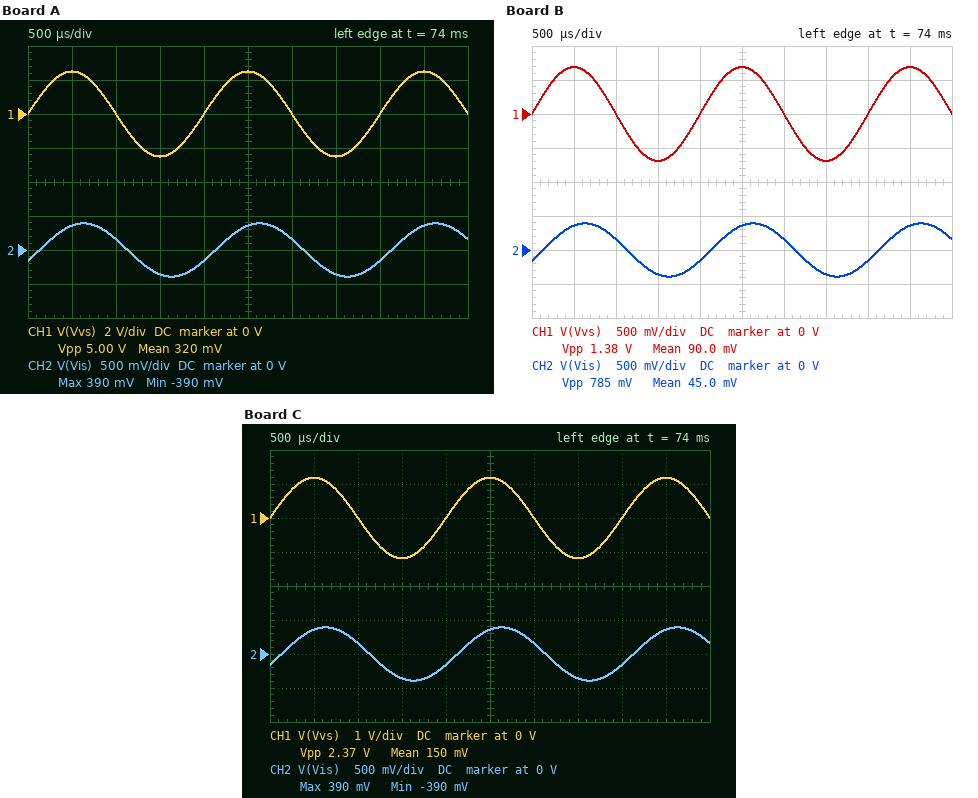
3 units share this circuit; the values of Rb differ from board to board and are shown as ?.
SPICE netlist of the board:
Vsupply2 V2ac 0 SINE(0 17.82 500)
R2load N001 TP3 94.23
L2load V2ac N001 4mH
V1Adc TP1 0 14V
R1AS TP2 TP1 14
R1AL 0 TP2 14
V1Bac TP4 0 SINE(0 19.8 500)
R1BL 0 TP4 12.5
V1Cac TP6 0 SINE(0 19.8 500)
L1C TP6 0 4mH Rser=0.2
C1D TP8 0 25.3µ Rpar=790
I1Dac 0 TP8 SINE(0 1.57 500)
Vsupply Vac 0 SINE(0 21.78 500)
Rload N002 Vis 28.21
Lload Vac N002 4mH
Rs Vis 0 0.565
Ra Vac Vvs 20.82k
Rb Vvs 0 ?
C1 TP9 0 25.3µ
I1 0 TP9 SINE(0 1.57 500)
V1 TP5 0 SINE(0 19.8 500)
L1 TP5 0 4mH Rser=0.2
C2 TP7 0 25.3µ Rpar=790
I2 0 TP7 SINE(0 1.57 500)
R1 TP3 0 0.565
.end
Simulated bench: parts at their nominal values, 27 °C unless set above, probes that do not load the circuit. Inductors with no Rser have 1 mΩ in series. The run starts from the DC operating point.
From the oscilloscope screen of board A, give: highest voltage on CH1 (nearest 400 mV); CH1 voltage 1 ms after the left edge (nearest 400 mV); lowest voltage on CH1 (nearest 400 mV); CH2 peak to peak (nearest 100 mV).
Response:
2.4 V
0 V
-2.4 V
800 mV
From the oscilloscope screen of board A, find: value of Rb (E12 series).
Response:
2.7 kΩ
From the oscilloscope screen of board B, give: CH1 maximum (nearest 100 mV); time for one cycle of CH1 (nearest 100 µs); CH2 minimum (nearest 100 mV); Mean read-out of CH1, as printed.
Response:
700 mV
2.0 ms
-400 mV
90.0 mV
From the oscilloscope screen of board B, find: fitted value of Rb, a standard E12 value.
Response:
680 Ω
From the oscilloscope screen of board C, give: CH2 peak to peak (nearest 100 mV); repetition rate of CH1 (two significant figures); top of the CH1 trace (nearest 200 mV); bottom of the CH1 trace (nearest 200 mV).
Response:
800 mV
500 Hz
1.2 V
-1.2 V
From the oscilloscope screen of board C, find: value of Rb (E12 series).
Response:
1.2 kΩ
